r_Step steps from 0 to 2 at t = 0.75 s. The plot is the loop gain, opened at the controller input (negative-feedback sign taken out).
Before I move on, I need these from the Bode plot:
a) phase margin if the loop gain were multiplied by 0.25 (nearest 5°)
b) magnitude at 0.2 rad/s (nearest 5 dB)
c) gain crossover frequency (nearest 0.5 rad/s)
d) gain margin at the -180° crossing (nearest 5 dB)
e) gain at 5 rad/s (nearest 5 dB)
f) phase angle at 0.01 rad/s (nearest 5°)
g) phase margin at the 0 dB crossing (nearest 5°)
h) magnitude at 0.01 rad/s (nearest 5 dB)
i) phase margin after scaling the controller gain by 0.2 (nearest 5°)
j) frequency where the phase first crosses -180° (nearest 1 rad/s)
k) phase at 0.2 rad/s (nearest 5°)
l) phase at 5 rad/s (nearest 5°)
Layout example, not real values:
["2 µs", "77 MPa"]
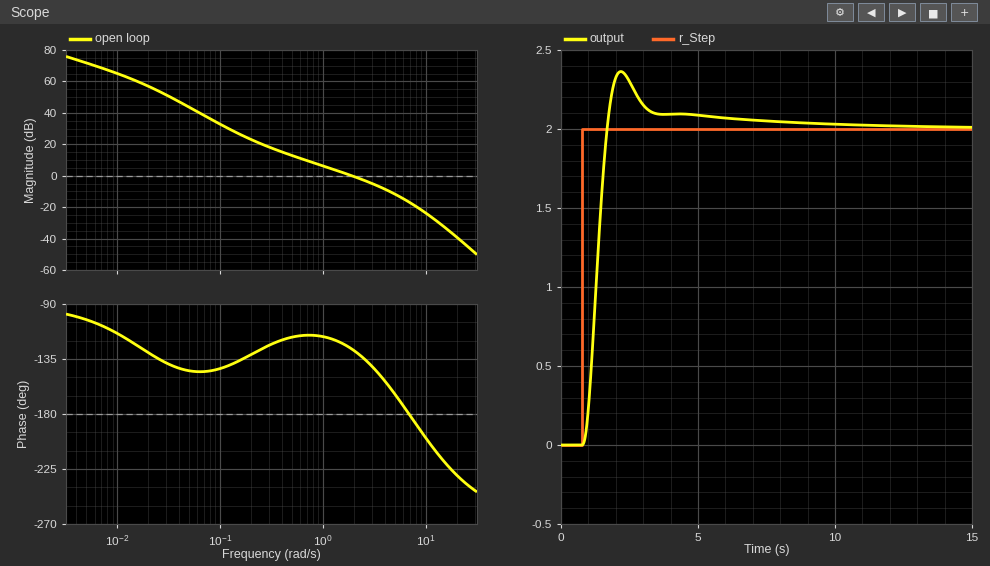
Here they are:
["65°", "25 dB", "2.0 rad/s", "15 dB", "-10 dB", "-115°", "55°", "65 dB", "60°", "7 rad/s", "-130°", "-165°"]
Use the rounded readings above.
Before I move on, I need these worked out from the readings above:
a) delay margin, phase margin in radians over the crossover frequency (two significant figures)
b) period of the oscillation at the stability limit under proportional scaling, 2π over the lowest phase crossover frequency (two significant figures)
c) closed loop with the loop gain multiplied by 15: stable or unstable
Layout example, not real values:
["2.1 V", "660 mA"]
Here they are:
["0.48 s", "0.90 s", "unstable"]
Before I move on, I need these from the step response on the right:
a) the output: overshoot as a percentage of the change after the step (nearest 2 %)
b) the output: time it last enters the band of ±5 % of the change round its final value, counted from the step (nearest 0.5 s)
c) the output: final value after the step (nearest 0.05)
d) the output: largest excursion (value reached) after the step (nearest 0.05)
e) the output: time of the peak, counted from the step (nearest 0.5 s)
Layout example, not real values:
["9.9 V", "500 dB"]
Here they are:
["18 %", "2.5 s", "2.00", "2.35", "1.5 s"]
